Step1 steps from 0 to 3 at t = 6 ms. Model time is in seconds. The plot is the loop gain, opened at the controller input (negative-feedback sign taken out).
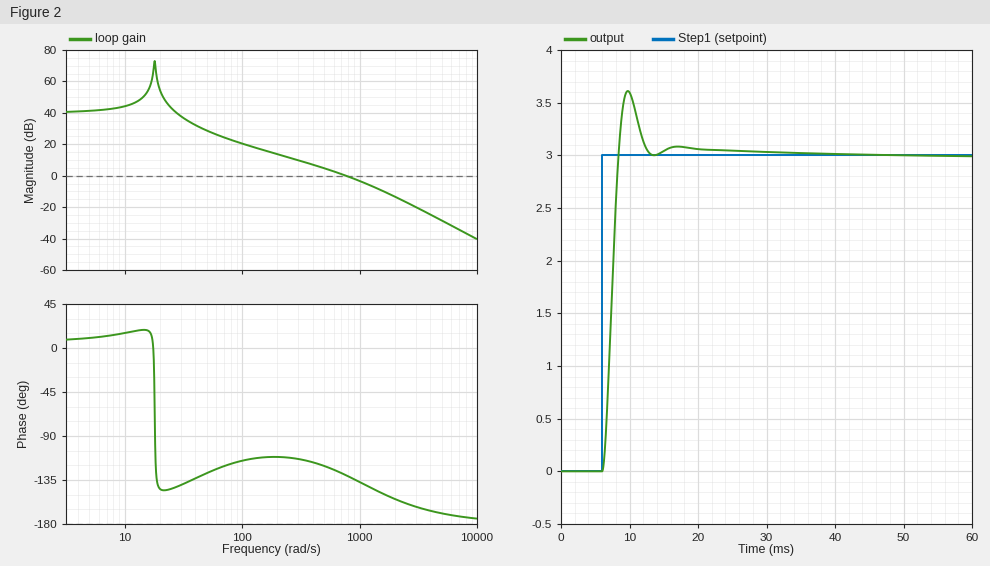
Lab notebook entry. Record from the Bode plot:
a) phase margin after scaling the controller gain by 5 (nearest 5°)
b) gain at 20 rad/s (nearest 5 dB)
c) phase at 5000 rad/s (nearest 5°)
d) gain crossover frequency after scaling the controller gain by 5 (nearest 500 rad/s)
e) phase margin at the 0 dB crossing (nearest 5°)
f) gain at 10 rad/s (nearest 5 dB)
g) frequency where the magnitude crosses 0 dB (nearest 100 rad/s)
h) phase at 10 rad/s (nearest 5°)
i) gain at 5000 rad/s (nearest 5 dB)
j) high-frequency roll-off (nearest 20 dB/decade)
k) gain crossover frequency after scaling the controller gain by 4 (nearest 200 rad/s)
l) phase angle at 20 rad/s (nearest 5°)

25°
55 dB
-170°
2000 rad/s
50°
45 dB
800 rad/s
15°
-30 dB
-40 dB/decade
1800 rad/s
-145°
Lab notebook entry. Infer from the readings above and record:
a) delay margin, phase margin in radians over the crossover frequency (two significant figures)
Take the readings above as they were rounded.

0.0011 s
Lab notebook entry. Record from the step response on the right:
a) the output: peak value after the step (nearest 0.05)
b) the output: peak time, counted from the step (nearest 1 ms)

3.60
4 ms
